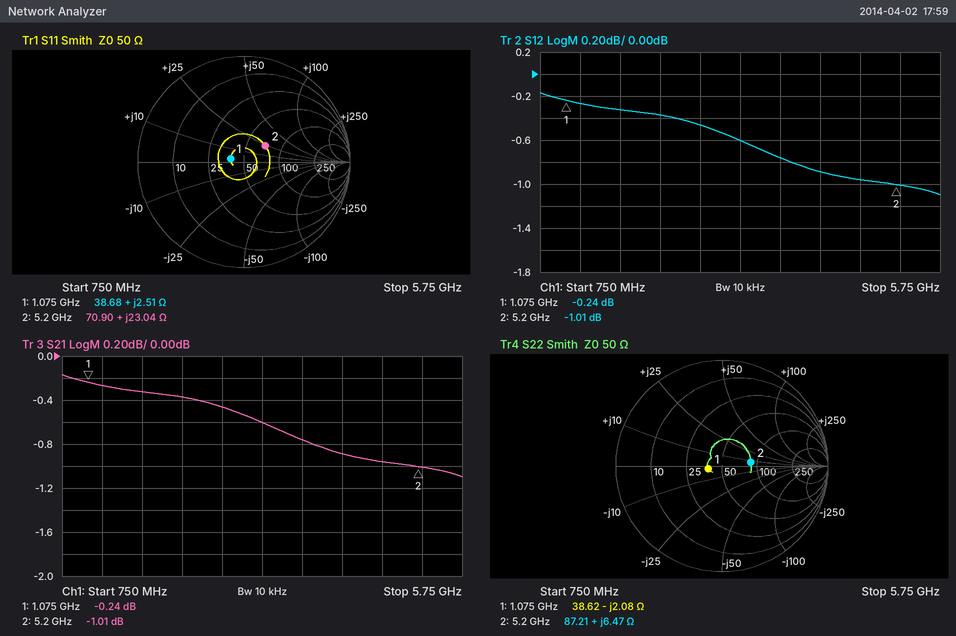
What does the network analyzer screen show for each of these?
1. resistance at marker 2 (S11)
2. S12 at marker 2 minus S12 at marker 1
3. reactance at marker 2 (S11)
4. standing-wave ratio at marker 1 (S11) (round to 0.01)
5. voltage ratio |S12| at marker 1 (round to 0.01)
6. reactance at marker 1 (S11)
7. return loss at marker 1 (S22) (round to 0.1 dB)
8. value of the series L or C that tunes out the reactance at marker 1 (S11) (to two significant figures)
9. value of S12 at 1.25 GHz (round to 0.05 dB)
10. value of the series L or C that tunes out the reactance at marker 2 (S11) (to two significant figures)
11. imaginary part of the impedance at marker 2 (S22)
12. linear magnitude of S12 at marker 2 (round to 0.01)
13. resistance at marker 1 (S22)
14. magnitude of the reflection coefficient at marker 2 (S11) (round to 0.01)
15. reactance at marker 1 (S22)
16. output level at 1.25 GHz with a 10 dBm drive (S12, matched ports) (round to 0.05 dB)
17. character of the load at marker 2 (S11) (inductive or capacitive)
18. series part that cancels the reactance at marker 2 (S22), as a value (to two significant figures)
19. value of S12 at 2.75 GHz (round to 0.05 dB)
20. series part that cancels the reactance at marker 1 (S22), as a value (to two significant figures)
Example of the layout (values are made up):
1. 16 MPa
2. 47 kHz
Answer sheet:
1. 70.90 Ω
2. -0.77 dB
3. +23.04 Ω
4. 1.30
5. 0.97
6. +2.51 Ω
7. 17.7 dB
8. 59 pF
9. -0.25 dB
10. 1.3 pF
11. +6.47 Ω
12. 0.89
13. 38.62 Ω
14. 0.25
15. -2.08 Ω
16. 9.75 dBm
17. inductive
18. 4.7 pF
19. -0.45 dB
20. 310 pH
